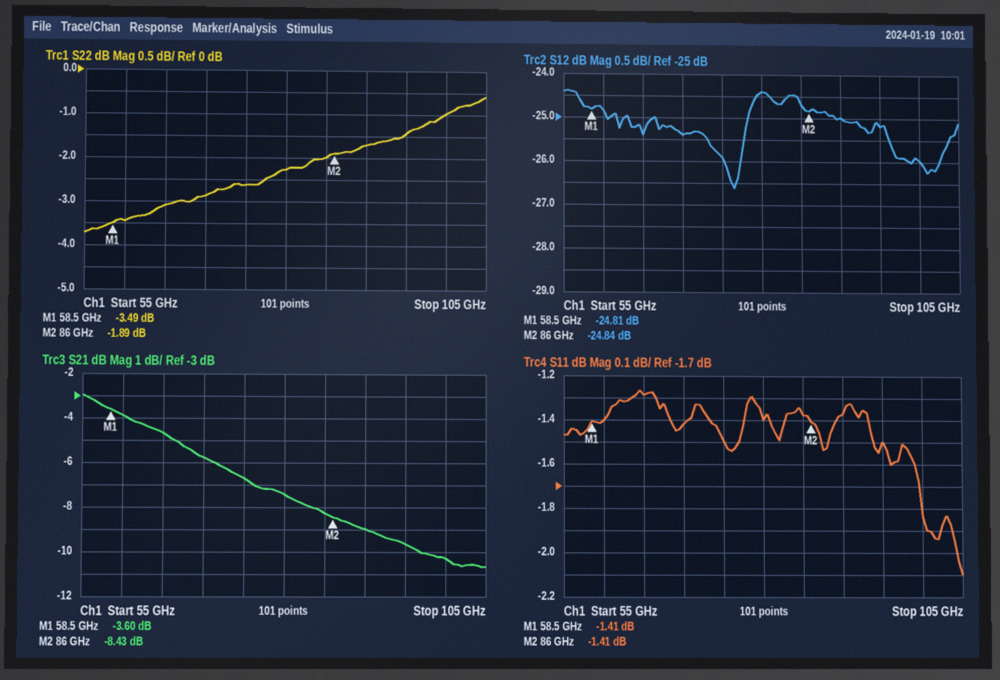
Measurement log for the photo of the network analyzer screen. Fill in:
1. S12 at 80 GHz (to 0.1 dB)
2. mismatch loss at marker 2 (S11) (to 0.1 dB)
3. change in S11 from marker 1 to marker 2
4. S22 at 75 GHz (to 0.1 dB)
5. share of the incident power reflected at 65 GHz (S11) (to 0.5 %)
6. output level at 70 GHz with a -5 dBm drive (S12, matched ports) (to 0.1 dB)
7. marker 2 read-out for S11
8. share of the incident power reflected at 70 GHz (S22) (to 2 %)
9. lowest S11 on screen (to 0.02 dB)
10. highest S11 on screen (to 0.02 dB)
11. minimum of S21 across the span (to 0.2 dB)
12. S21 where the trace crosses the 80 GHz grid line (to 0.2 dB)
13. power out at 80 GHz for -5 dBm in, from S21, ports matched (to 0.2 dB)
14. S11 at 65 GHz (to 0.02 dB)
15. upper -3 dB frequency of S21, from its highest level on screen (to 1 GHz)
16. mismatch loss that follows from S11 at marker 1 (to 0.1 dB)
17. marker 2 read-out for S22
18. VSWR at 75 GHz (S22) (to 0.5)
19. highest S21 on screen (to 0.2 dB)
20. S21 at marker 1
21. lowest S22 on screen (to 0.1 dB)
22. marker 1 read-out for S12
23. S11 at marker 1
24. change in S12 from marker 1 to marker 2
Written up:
-24.4 dB
5.6 dB
0.00 dB
-2.6 dB
74.5 %
-30.4 dBm
-1.41 dB
52 %
-2.10 dB
-1.26 dB
-10.6 dB
-7.4 dB
-12.4 dBm
-1.28 dB
71 GHz
5.6 dB
-1.89 dB
6.5
-3.0 dB
-3.60 dB
-3.7 dB
-24.81 dB
-1.41 dB
-0.03 dB
